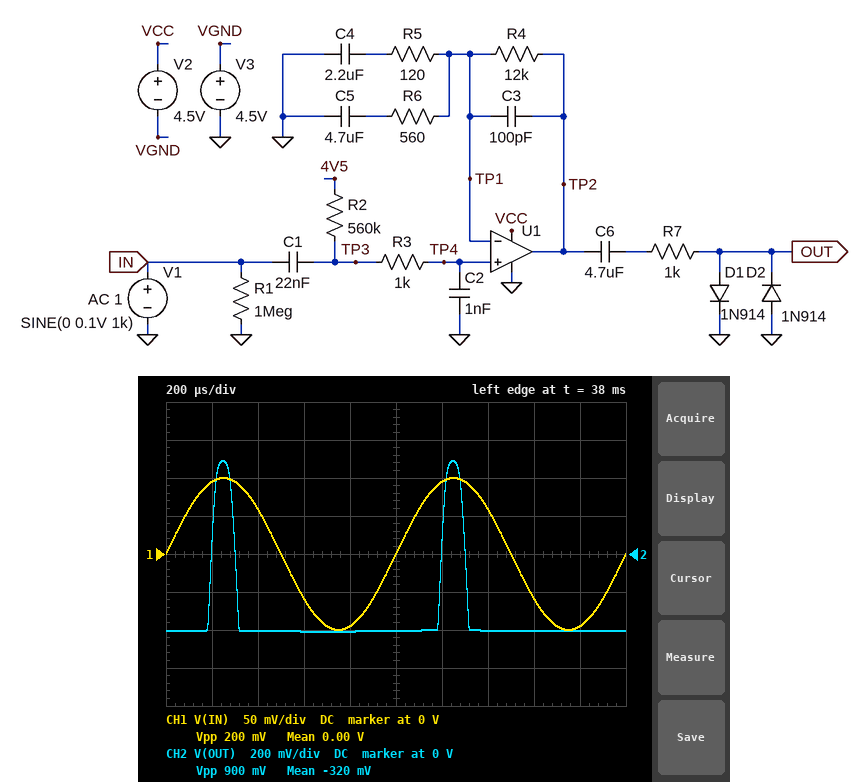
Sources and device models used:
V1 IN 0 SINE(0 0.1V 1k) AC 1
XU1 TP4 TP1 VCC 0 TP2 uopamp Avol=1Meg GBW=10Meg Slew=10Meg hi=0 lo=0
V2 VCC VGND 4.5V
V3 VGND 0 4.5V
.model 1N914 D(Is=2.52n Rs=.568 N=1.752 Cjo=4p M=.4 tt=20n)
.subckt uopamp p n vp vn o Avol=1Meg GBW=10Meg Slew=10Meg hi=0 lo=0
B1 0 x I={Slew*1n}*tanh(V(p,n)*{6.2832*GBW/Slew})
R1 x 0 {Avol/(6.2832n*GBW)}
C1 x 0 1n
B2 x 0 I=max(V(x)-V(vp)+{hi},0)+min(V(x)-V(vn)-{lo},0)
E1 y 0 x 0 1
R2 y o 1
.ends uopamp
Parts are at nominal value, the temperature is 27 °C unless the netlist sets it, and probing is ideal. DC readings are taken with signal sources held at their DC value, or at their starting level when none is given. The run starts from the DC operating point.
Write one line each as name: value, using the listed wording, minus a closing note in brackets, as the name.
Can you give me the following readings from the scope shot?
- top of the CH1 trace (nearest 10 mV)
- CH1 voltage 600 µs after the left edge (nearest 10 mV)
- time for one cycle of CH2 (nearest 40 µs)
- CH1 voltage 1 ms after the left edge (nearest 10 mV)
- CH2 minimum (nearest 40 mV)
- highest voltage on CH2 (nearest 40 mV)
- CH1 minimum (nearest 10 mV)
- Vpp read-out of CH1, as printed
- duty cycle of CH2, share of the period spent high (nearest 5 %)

top of the CH1 trace: 100 mV
CH1 voltage 600 µs after the left edge: -60 mV
time for one cycle of CH2: 1.00 ms
CH1 voltage 1 ms after the left edge: 0 V
CH2 minimum: -400 mV
highest voltage on CH2: 480 mV
CH1 minimum: -100 mV
Vpp read-out of CH1, as printed: 200 mV
duty cycle of CH2, share of the period spent high: 10 %
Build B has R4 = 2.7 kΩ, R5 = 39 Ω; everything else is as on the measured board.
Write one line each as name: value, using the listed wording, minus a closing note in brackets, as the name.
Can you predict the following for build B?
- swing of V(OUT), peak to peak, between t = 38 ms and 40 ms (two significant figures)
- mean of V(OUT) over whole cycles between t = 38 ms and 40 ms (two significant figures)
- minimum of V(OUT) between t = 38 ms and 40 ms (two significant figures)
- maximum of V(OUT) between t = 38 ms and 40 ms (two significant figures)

swing of V(OUT), peak to peak, between t = 38 ms and 40 ms: 740 mV
mean of V(OUT) over whole cycles between t = 38 ms and 40 ms: -170 mV
minimum of V(OUT) between t = 38 ms and 40 ms: -260 mV
maximum of V(OUT) between t = 38 ms and 40 ms: 480 mV
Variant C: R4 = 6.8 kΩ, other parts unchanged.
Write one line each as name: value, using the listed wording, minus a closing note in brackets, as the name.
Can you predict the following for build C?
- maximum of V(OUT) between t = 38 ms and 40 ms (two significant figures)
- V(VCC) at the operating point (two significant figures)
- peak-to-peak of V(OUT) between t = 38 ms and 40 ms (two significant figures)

maximum of V(OUT) between t = 38 ms and 40 ms: 430 mV
V(VCC) at the operating point: 9.0 V
peak-to-peak of V(OUT) between t = 38 ms and 40 ms: 800 mV
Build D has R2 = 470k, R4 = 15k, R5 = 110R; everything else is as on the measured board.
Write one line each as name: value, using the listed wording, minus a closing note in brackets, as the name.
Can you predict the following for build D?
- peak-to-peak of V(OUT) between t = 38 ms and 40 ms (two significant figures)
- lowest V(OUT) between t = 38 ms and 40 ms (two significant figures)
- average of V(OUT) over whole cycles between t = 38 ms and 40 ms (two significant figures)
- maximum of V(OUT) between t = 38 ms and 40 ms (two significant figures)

peak-to-peak of V(OUT) between t = 38 ms and 40 ms: 930 mV
lowest V(OUT) between t = 38 ms and 40 ms: -420 mV
average of V(OUT) over whole cycles between t = 38 ms and 40 ms: -330 mV
maximum of V(OUT) between t = 38 ms and 40 ms: 510 mV
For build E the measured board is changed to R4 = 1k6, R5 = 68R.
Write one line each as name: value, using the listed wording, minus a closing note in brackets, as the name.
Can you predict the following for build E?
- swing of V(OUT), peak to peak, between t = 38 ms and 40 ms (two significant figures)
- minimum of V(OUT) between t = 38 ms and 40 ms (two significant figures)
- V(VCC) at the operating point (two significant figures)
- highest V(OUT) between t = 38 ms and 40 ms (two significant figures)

swing of V(OUT), peak to peak, between t = 38 ms and 40 ms: 530 mV
minimum of V(OUT) between t = 38 ms and 40 ms: -100 mV
V(VCC) at the operating point: 9.0 V
highest V(OUT) between t = 38 ms and 40 ms: 430 mV
